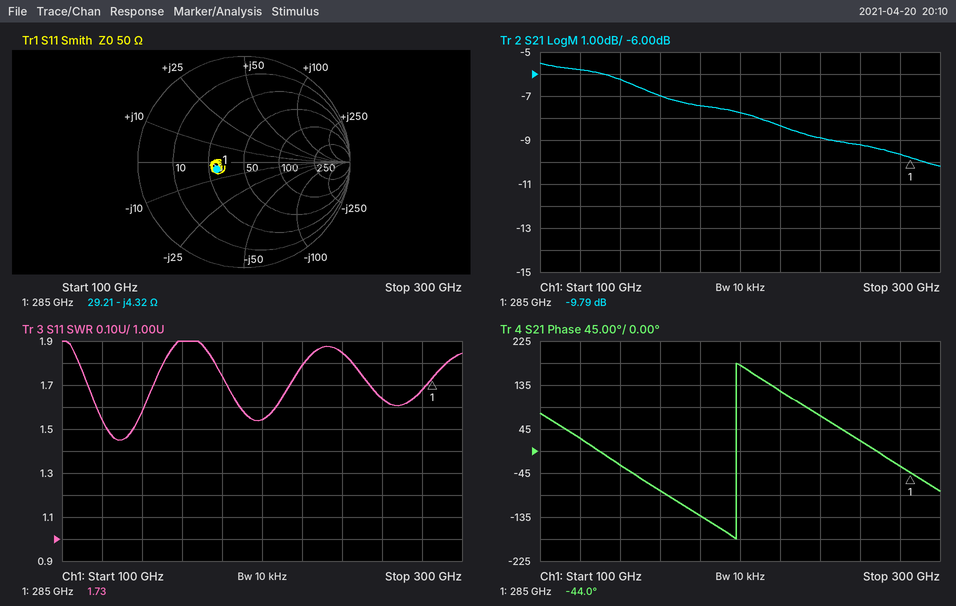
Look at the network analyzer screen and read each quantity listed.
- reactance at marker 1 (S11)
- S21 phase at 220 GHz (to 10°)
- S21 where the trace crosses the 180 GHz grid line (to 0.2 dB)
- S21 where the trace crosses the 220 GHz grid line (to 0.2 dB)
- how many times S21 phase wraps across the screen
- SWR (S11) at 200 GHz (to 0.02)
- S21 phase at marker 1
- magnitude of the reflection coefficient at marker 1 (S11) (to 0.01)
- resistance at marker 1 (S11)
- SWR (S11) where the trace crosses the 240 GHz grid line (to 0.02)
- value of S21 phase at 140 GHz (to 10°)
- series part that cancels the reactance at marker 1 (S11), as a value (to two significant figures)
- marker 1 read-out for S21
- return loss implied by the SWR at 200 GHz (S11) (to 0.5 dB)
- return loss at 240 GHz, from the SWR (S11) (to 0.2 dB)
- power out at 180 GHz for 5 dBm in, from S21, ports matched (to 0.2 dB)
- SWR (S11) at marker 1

-4.32 Ω
120°
-7.4 dB
-8.4 dB
1
1.54
-44.0°
0.27
29.21 Ω
1.84
-30°
2.4 pH
-9.79 dB
13.5 dB
10.6 dB
-2.4 dBm
1.73
